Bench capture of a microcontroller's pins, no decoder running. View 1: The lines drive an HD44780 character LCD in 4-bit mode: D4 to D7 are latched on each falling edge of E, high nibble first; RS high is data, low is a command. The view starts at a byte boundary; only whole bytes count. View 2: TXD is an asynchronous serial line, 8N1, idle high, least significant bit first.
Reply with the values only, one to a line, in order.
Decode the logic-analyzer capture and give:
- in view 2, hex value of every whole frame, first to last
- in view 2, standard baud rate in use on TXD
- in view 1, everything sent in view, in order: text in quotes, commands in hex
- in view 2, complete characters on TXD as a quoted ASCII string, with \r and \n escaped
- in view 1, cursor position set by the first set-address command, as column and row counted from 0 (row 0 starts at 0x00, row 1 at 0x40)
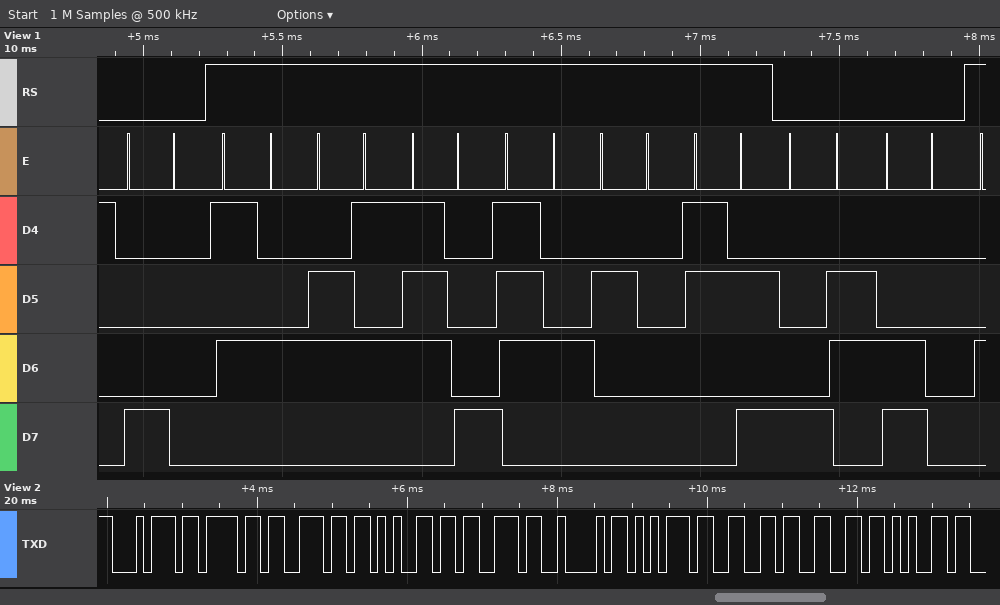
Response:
74 6F 6E 65 73 42 75 66 66 65
9600 baud
0x80 "Text :" 0x86 0xC0
"tonesBuffe"
column 0, row 0
